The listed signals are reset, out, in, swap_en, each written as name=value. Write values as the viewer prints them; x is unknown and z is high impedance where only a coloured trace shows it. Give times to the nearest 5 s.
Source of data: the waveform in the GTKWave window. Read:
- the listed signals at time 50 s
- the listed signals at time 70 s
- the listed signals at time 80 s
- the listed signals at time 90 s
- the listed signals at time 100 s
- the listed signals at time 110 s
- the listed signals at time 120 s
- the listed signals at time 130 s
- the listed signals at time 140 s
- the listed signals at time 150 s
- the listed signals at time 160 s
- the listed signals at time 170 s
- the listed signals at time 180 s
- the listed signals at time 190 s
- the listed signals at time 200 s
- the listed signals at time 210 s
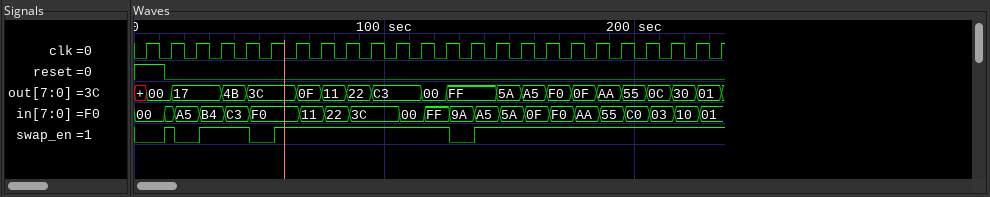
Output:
reset=0, out=3C, in=F0, swap_en=0
reset=0, out=0F, in=11, swap_en=1
reset=0, out=11, in=22, swap_en=1
reset=0, out=22, in=3C, swap_en=1
reset=0, out=C3, in=3C, swap_en=1
reset=0, out=C3, in=00, swap_en=1
reset=0, out=00, in=FF, swap_en=1
reset=0, out=FF, in=9A, swap_en=0
reset=0, out=FF, in=A5, swap_en=1
reset=0, out=5A, in=5A, swap_en=1
reset=0, out=A5, in=0F, swap_en=1
reset=0, out=F0, in=F0, swap_en=1
reset=0, out=0F, in=AA, swap_en=1
reset=0, out=AA, in=55, swap_en=1
reset=0, out=55, in=C0, swap_en=1
reset=0, out=0C, in=03, swap_en=1
